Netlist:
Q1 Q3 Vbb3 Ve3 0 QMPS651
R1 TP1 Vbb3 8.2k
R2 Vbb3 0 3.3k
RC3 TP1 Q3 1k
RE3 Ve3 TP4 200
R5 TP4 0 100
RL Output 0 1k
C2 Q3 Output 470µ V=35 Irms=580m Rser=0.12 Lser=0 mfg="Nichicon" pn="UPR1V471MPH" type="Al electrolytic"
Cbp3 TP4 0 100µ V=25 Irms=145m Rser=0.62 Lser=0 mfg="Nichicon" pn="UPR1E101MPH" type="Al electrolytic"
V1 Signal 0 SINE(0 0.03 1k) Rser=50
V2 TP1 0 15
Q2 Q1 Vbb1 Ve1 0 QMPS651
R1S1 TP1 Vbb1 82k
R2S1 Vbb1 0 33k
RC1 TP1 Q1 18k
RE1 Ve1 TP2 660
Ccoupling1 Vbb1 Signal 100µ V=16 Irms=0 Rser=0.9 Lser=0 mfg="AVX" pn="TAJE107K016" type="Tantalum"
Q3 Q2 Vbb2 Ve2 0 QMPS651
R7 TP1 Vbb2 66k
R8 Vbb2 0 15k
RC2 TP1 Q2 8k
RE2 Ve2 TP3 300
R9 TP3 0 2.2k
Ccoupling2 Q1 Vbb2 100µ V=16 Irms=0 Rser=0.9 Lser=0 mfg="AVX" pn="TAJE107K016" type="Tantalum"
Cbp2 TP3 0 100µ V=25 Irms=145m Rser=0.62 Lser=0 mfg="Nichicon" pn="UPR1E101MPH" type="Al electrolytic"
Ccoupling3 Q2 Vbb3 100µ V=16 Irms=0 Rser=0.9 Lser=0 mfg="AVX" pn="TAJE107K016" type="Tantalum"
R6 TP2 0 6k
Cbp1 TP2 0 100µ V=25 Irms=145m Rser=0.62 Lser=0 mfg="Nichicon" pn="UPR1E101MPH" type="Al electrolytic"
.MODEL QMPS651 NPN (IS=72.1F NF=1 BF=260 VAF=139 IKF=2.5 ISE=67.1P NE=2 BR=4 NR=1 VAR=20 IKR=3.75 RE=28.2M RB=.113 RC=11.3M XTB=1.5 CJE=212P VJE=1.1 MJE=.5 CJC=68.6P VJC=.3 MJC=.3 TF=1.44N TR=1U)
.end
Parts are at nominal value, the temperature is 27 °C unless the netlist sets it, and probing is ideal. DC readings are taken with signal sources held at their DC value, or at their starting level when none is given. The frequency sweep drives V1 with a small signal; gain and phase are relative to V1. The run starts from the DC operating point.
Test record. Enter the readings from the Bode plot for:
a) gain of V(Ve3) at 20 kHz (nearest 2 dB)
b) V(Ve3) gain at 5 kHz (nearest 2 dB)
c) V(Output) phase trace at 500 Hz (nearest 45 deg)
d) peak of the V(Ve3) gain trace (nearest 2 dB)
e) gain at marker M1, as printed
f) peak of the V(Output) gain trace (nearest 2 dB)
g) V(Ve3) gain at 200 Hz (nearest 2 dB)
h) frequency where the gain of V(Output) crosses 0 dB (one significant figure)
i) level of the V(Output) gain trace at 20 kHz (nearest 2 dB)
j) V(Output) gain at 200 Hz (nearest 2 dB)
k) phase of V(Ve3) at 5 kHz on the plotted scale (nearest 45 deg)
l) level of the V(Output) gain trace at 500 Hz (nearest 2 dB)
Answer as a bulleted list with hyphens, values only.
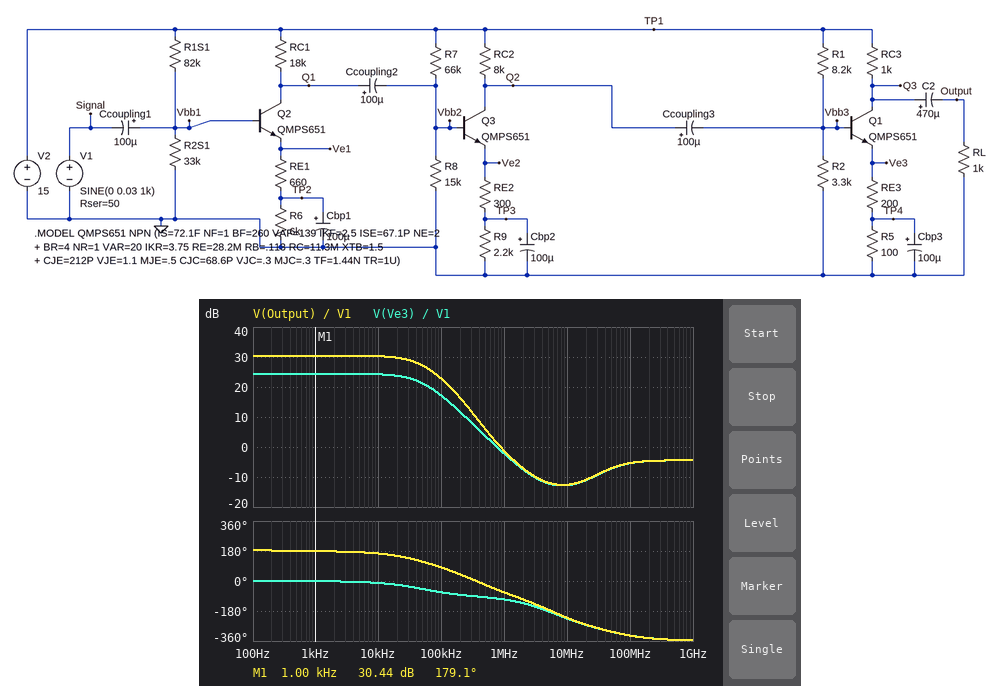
- 24 dB
- 24 dB
- 180 deg
- 24 dB
- 30.44 dB
- 30 dB
- 24 dB
- 900 kHz
- 30 dB
- 30 dB
- 0 deg
- 30 dB
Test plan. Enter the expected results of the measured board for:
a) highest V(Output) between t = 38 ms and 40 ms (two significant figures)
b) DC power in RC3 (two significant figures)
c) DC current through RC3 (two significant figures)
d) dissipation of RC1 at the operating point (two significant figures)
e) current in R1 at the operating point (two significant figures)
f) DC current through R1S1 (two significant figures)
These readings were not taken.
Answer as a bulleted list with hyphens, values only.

- 2.9 V
- 130 mW
- 11 mA
- 4.9 mW
- 1.3 mA
- 130 µA
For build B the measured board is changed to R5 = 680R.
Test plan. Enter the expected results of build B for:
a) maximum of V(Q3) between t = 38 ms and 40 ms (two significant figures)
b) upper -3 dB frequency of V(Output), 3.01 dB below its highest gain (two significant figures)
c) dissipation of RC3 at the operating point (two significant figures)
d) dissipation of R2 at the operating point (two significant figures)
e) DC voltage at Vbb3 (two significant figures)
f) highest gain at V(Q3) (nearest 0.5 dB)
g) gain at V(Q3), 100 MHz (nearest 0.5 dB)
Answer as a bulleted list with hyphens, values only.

- 13 V
- 94 kHz
- 16 mW
- 5.4 mW
- 4.2 V
- 40.5 dB
- -4.5 dB
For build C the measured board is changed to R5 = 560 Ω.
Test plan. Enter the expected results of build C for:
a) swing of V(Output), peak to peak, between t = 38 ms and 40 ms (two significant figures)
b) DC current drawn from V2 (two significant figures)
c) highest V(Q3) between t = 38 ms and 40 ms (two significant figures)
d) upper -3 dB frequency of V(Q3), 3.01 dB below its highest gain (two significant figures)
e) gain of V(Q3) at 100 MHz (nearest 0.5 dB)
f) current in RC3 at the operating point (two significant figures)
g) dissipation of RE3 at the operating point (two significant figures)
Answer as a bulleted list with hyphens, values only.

- 5.2 V
- 7.6 mA
- 13 V
- 94 kHz
- -4.5 dB
- 4.7 mA
- 4.4 mW
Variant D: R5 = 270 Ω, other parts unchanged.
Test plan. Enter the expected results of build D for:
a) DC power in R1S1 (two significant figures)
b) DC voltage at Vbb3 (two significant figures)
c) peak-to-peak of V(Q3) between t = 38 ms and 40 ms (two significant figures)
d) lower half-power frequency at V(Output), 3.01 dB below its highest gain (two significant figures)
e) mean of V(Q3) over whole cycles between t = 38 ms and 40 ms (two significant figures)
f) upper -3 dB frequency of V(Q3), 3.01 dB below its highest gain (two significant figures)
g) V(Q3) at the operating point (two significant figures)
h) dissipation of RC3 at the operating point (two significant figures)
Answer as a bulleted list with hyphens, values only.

- 1.4 mW
- 4.2 V
- 6.0 V
- 13 Hz
- 7.6 V
- 93 kHz
- 7.5 V
- 56 mW
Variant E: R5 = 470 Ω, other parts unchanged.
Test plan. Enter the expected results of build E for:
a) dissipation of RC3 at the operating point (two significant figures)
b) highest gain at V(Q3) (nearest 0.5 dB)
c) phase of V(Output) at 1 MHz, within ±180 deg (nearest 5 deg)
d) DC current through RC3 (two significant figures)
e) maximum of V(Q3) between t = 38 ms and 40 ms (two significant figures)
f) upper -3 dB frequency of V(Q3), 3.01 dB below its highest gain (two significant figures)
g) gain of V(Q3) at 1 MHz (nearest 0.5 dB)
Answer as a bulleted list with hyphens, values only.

- 28 mW
- 40.5 dB
- 40 deg
- 5.3 mA
- 12 V
- 94 kHz
- 19.0 dB
